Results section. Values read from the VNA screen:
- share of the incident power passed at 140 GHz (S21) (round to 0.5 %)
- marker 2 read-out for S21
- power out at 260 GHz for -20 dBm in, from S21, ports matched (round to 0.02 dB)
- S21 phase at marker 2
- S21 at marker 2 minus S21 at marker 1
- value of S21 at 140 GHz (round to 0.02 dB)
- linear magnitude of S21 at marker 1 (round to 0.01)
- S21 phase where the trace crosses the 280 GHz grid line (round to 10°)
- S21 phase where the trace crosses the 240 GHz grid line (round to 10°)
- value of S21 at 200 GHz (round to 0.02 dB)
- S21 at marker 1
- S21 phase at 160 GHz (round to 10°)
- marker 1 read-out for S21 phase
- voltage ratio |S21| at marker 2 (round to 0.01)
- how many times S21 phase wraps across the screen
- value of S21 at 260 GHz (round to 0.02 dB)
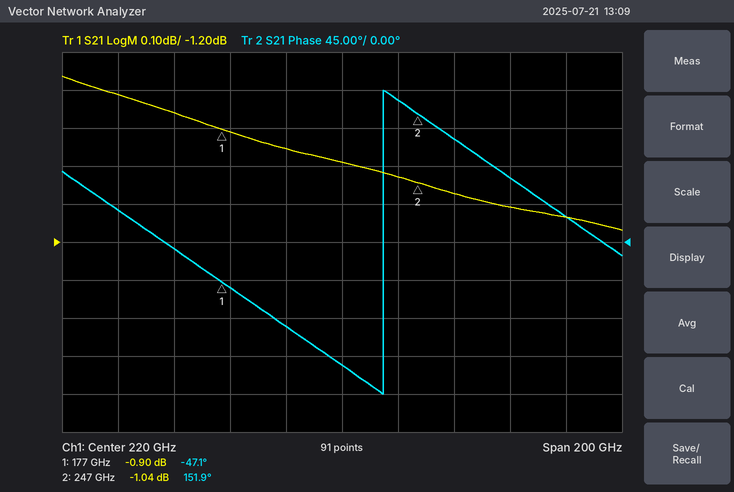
83.0 %
-1.04 dB
-21.08 dBm
151.9°
-0.14 dB
-0.82 dB
0.90
80°
170°
-0.96 dB
-0.90 dB
-10°
-47.1°
0.89
1
-1.08 dB
